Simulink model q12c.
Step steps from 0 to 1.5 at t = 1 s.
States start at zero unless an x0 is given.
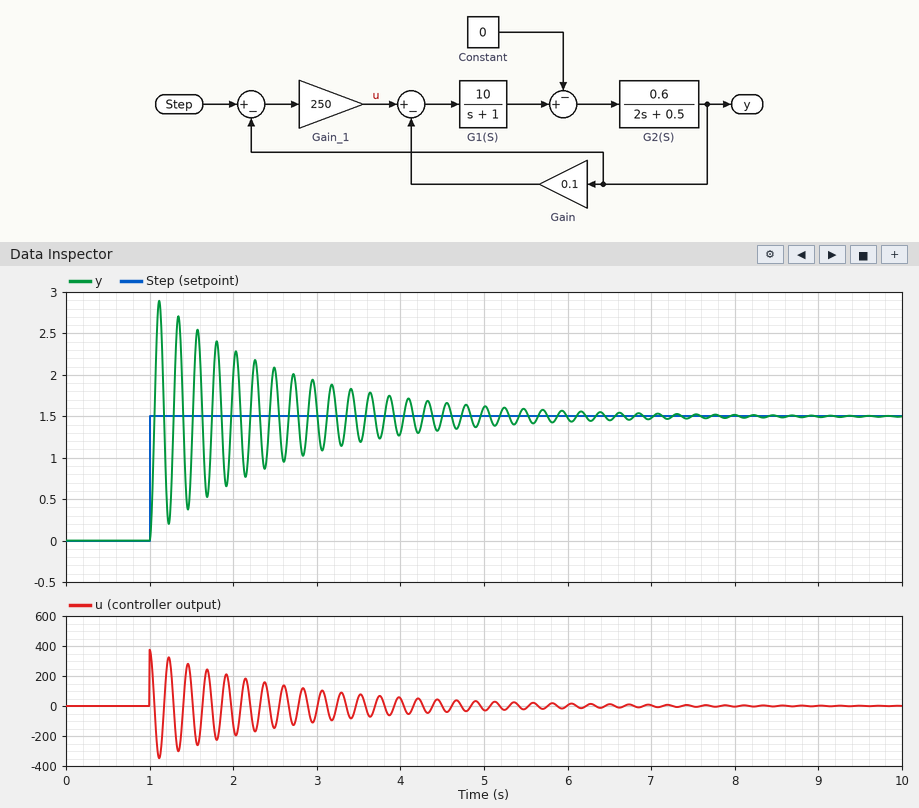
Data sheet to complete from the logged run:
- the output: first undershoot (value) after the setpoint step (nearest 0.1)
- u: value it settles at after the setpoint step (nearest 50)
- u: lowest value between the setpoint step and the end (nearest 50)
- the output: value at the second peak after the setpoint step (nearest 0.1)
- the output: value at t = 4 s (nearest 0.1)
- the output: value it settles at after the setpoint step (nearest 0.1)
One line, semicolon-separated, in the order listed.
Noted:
0.2; 0; -350; 2.7; 1.3; 1.5
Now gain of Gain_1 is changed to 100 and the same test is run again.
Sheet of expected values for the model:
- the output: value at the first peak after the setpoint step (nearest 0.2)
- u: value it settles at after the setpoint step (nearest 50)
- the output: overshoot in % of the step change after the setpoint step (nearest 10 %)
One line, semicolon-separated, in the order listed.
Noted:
2.8; 0; 90 %
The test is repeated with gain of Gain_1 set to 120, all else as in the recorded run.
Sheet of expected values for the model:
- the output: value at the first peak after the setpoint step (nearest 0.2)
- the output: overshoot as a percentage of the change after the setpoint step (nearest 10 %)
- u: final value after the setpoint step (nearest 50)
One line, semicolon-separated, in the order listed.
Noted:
2.8; 90 %; 0
